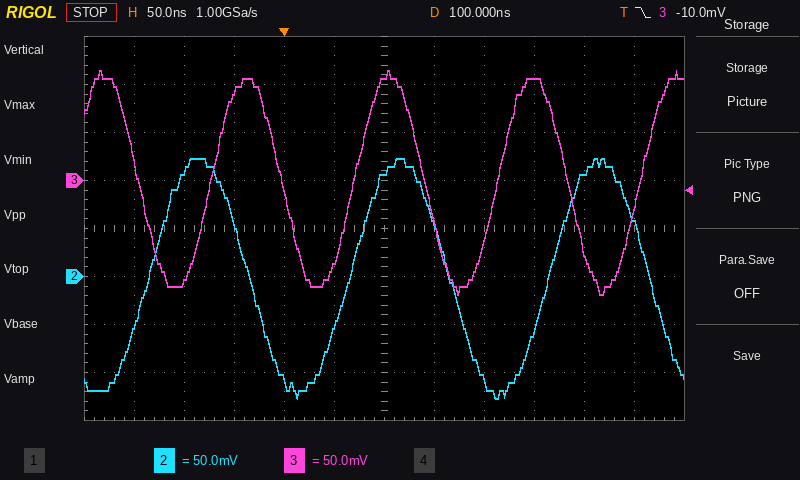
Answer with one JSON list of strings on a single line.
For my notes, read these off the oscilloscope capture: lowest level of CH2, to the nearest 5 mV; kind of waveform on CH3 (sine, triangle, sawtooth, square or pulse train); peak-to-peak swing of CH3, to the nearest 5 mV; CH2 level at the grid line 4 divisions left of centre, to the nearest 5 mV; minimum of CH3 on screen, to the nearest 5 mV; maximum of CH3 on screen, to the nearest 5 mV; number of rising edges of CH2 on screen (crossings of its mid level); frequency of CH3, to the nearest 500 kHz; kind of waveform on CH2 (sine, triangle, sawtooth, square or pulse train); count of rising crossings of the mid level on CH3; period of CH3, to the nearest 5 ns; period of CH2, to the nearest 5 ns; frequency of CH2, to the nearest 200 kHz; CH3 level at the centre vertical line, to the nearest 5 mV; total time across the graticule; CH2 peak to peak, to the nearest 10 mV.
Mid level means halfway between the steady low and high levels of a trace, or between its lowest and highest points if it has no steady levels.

["-125 mV", "sine", "235 mV", "110 mV", "-120 mV", "115 mV", "3", "7.0 MHz", "sine", "4", "145 ns", "200 ns", "5.0 MHz", "110 mV", "600 ns", "250 mV"]
